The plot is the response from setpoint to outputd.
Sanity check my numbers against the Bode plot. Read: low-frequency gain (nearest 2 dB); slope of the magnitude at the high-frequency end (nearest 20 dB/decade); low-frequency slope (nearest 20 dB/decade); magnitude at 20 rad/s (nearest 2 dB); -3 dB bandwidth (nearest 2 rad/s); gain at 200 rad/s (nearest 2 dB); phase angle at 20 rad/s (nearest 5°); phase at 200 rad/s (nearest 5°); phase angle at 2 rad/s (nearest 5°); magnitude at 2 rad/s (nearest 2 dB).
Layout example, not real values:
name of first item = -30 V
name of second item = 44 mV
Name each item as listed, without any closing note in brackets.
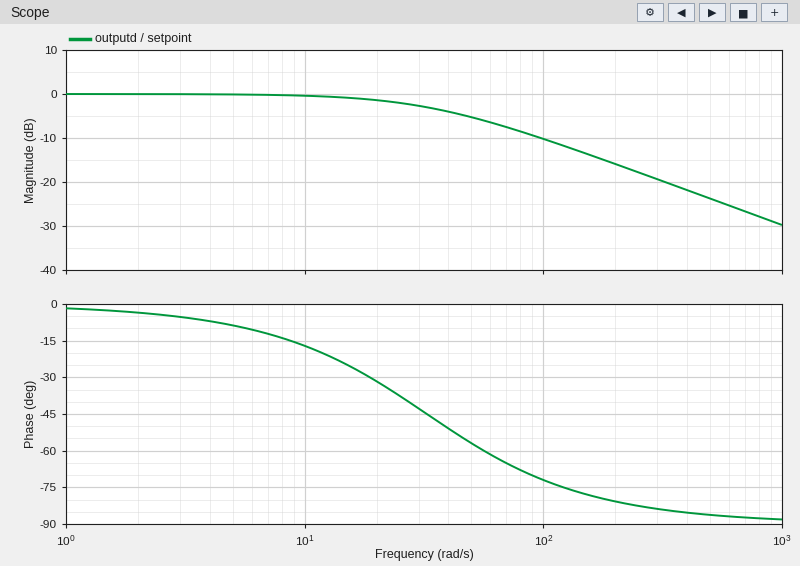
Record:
low-frequency gain = 0 dB
slope of the magnitude at the high-frequency end = -20 dB/decade
low-frequency slope = 0 dB/decade
magnitude at 20 rad/s = -2 dB
-3 dB bandwidth = 32 rad/s
gain at 200 rad/s = -16 dB
phase angle at 20 rad/s = -30°
phase at 200 rad/s = -80°
phase angle at 2 rad/s = -5°
magnitude at 2 rad/s = 0 dB
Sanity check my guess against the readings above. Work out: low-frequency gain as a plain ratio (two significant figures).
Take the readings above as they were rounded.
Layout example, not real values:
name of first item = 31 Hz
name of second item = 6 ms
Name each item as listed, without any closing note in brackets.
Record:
low-frequency gain as a plain ratio = 1.0
